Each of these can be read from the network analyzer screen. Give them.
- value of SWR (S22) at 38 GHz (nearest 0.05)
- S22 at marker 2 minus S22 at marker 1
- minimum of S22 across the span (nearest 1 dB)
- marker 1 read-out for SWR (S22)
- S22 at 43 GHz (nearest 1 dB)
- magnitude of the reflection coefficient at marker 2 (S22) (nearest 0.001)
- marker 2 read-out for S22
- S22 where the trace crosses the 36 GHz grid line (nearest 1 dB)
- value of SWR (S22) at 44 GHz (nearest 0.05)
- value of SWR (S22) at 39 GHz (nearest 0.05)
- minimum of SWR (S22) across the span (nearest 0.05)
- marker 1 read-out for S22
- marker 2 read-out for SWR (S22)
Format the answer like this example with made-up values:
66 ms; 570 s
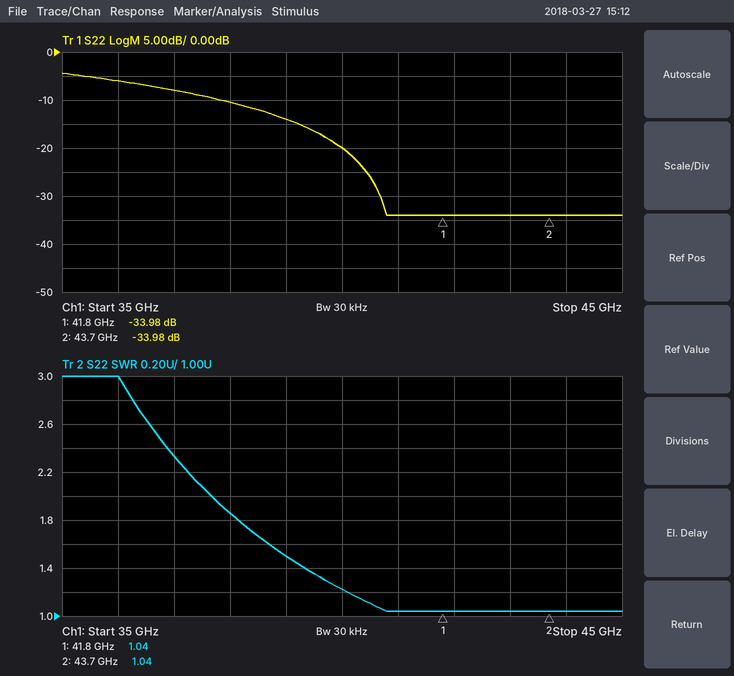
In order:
1.85; 0.00 dB; -34 dB; 1.04; -34 dB; 0.020; -33.98 dB; -6 dB; 1.05; 1.50; 1.05; -33.98 dB; 1.04
